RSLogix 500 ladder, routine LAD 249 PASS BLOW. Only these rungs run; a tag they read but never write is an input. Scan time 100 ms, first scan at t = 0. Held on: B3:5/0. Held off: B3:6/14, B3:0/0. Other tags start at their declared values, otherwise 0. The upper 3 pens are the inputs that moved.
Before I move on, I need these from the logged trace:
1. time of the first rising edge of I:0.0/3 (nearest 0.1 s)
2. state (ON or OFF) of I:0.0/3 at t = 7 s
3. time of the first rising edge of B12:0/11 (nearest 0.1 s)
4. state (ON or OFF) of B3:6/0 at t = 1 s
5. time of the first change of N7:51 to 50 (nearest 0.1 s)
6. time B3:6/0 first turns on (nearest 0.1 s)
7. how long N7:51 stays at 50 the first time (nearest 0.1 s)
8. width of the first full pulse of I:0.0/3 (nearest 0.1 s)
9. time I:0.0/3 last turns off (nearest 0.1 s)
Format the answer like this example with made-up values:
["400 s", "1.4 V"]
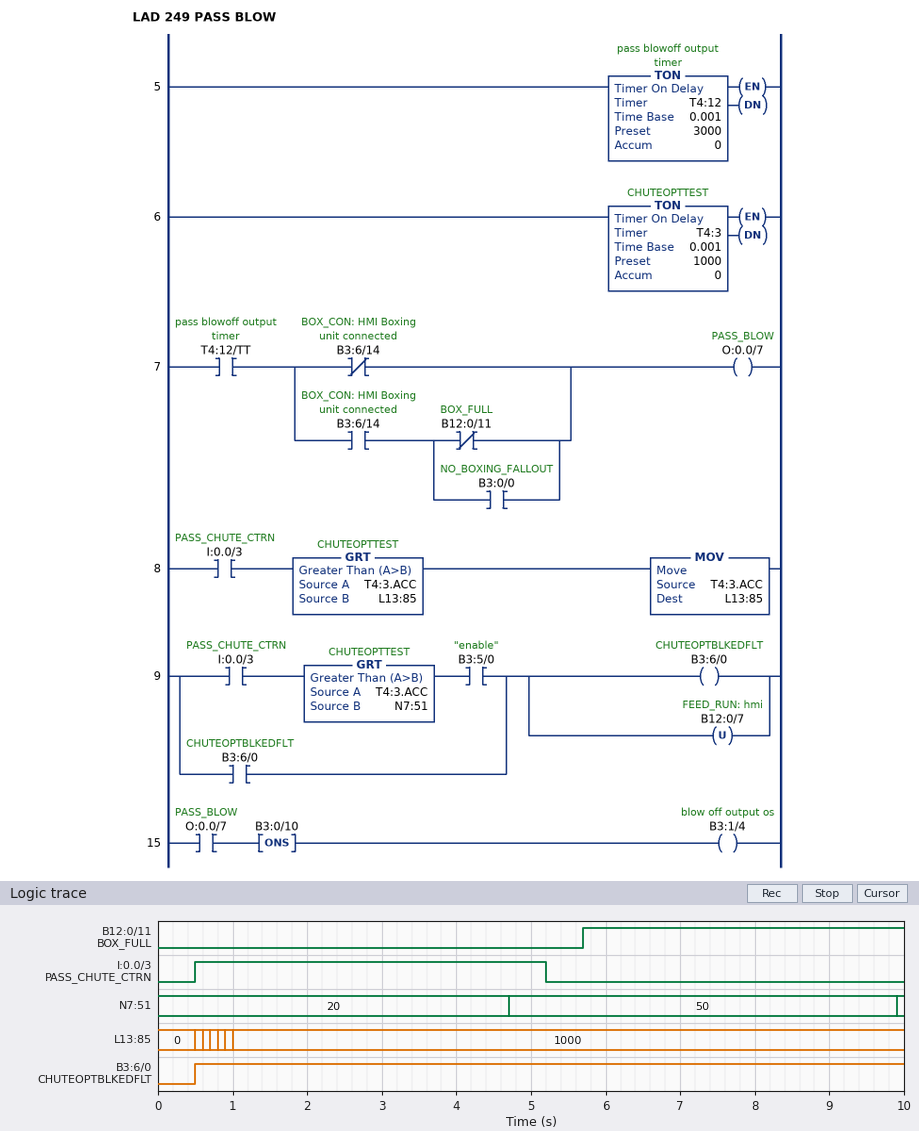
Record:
["0.5 s", "OFF", "5.7 s", "ON", "4.7 s", "0.5 s", "5.2 s", "4.7 s", "5.2 s"]
